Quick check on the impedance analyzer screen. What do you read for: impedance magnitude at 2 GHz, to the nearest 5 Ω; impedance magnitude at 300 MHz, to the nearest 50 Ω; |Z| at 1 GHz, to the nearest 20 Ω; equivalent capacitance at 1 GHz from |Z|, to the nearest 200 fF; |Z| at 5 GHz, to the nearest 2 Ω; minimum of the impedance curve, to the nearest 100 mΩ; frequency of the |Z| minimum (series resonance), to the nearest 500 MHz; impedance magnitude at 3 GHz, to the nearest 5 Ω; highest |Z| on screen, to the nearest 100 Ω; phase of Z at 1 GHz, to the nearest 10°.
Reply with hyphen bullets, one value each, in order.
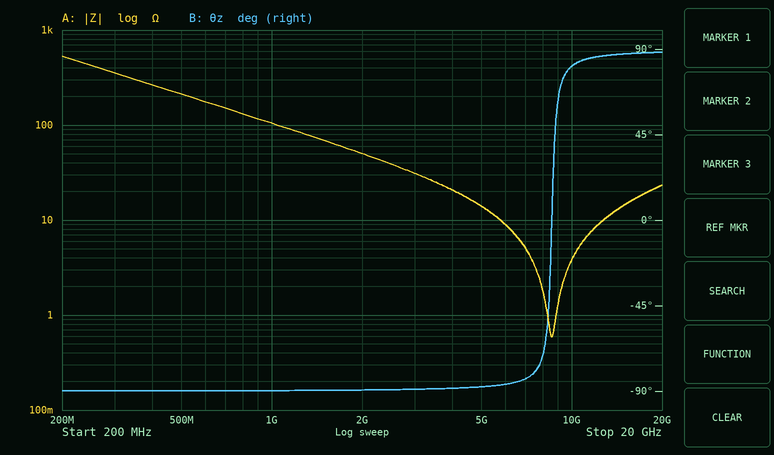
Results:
- 50 Ω
- 350 Ω
- 100 Ω
- 1.6 pF
- 14 Ω
- 600 mΩ
- 8.5 GHz
- 30 Ω
- 500 Ω
- -90°
